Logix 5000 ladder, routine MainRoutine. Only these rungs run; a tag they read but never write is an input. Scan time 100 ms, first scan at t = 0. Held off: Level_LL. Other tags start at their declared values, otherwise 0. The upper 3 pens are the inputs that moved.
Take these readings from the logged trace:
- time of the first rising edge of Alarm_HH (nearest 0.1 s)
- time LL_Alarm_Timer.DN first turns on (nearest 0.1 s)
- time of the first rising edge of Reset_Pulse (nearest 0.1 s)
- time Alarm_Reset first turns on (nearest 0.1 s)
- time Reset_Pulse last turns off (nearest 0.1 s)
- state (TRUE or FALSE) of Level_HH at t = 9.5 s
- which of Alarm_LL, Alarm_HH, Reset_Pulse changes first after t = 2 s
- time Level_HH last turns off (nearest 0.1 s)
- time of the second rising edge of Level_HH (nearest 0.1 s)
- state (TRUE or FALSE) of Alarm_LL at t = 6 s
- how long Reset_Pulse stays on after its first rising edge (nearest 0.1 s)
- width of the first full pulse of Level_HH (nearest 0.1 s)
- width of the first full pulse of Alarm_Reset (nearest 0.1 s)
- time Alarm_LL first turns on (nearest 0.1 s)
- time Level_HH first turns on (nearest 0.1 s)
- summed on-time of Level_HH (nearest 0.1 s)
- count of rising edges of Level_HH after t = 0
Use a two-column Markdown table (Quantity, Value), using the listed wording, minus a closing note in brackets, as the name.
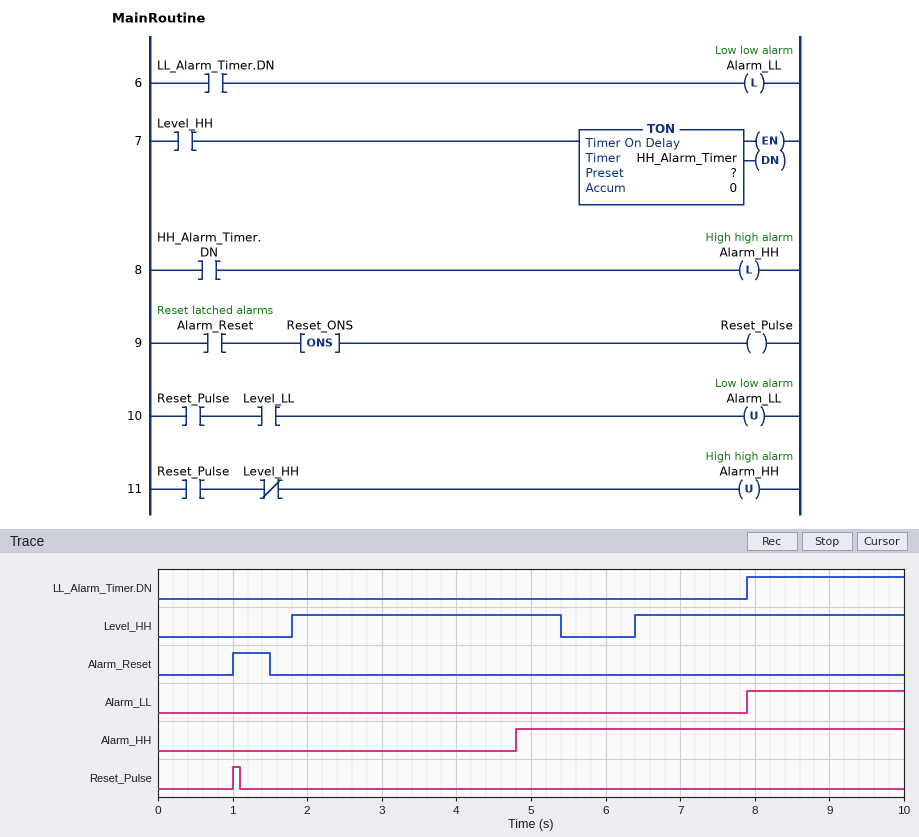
| Quantity | Value |
|---|---|
| time of the first rising edge of Alarm_HH | 4.8 s |
| time LL_Alarm_Timer.DN first turns on | 7.9 s |
| time of the first rising edge of Reset_Pulse | 1.0 s |
| time Alarm_Reset first turns on | 1.0 s |
| time Reset_Pulse last turns off | 1.1 s |
| state (TRUE or FALSE) of Level_HH at t = 9.5 s | TRUE |
| which of Alarm_LL, Alarm_HH, Reset_Pulse changes first after t = 2 s | Alarm_HH |
| time Level_HH last turns off | 5.4 s |
| time of the second rising edge of Level_HH | 6.4 s |
| state (TRUE or FALSE) of Alarm_LL at t = 6 s | FALSE |
| how long Reset_Pulse stays on after its first rising edge | 0.1 s |
| width of the first full pulse of Level_HH | 3.6 s |
| width of the first full pulse of Alarm_Reset | 0.5 s |
| time Alarm_LL first turns on | 7.9 s |
| time Level_HH first turns on | 1.8 s |
| summed on-time of Level_HH | 7.2 s |
| count of rising edges of Level_HH after t = 0 | 2 |
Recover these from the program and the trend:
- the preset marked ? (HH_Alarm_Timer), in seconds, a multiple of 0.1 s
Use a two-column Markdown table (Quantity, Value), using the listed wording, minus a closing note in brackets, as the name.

| Quantity | Value |
|---|---|
| the preset marked ? (HH_Alarm_Timer), in seconds, a multiple of 0.1 s | 3.0 s |
